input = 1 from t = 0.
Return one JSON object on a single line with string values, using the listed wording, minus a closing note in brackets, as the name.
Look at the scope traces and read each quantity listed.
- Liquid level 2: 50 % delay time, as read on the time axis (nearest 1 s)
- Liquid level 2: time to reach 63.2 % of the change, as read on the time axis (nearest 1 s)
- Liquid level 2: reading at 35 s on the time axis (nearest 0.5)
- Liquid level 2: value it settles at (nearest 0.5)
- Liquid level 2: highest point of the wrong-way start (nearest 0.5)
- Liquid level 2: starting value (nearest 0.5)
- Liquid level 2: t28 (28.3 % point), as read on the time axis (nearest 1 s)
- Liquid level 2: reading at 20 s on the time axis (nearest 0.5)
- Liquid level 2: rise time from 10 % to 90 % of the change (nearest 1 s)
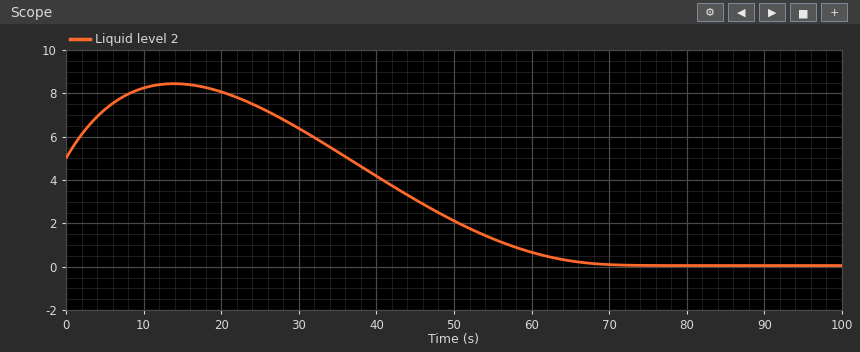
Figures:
{"Liquid level 2: 50 % delay time, as read on the time axis": "48 s", "Liquid level 2: time to reach 63.2 % of the change, as read on the time axis": "51 s", "Liquid level 2: reading at 35 s on the time axis": "5.5", "Liquid level 2: value it settles at": "0.0", "Liquid level 2: highest point of the wrong-way start": "8.5", "Liquid level 2: starting value": "5.0", "Liquid level 2: t28 (28.3 % point), as read on the time axis": "43 s", "Liquid level 2: reading at 20 s on the time axis": "8.0", "Liquid level 2: rise time from 10 % to 90 % of the change": "23 s"}
